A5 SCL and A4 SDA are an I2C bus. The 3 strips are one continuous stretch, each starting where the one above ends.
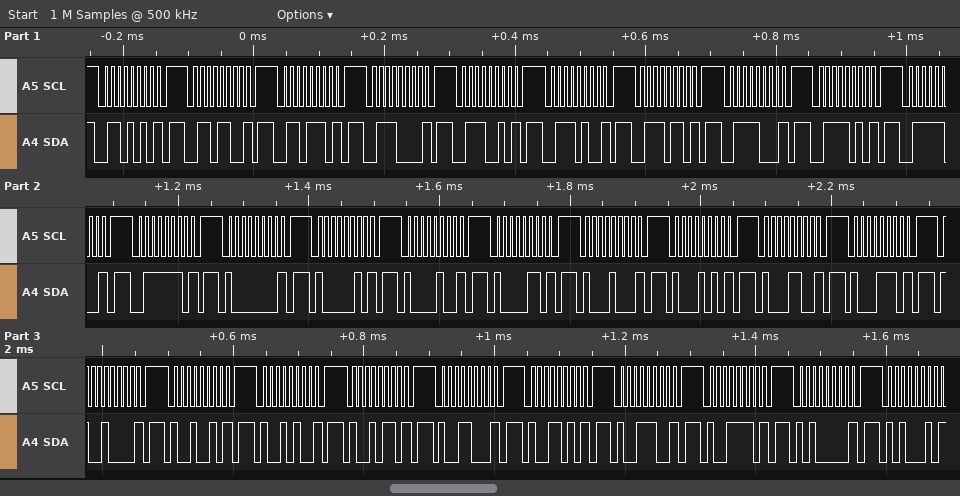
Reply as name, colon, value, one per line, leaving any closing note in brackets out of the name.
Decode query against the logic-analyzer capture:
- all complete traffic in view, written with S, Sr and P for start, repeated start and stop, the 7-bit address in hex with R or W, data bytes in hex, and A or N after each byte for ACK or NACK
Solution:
all complete traffic in view, written with S, Sr and P for start, repeated start and stop, the 7-bit address in hex with R or W, data bytes in hex, and A or N after each byte for ACK or NACK: S 35W N P S 36W N P S 37W N P S 38W N P S 39W N P S 3AW N P S 3BW N P S 3CW N P S 3DW N P S 3EW N P S 3FW N P S 40W N P S 41W N P S 42W N P S 43W N P S 44W N P S 45W N P S 46W N P S 47W N P S 48W N P S 49W N P S 4AW N P S 4BW N P S 4CW N P S 4DW N P S 4EW N P S 4FW N P S 50W N P S 51W N
